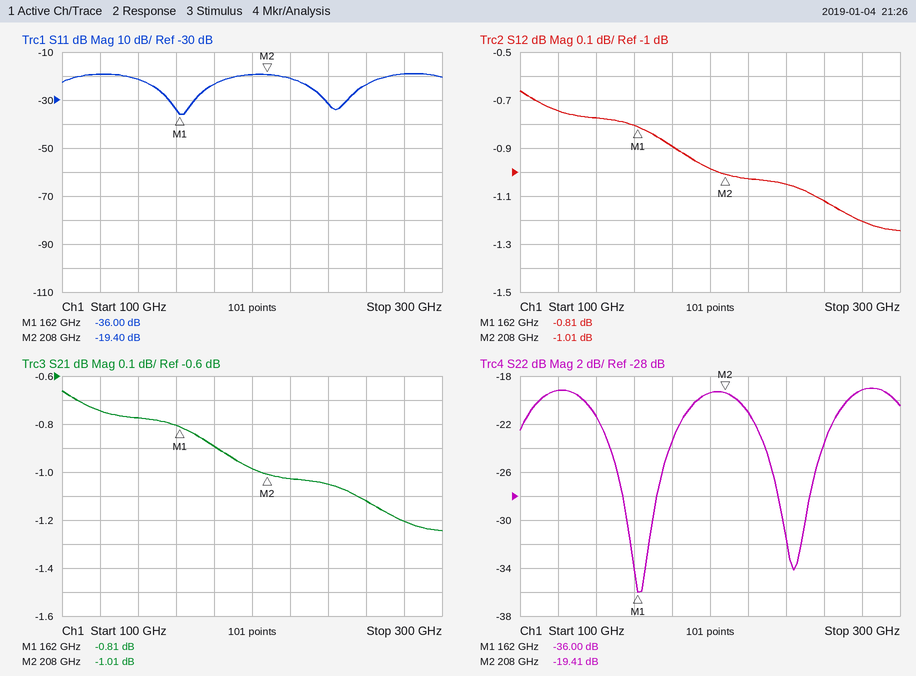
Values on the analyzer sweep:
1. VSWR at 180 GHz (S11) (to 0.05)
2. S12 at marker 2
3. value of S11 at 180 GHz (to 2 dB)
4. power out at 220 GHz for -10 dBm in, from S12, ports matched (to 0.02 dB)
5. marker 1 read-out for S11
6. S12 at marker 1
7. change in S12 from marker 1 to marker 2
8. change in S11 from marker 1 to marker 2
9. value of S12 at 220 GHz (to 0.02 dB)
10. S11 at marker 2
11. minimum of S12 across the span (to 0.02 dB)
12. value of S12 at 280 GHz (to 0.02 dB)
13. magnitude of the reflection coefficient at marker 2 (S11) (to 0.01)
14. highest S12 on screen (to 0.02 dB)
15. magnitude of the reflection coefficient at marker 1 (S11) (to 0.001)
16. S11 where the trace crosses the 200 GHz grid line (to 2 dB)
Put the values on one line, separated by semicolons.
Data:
1.15; -1.01 dB; -24 dB; -11.02 dBm; -36.00 dB; -0.81 dB; -0.20 dB; 16.60 dB; -1.02 dB; -19.40 dB; -1.24 dB; -1.20 dB; 0.11; -0.66 dB; 0.016; -20 dB
